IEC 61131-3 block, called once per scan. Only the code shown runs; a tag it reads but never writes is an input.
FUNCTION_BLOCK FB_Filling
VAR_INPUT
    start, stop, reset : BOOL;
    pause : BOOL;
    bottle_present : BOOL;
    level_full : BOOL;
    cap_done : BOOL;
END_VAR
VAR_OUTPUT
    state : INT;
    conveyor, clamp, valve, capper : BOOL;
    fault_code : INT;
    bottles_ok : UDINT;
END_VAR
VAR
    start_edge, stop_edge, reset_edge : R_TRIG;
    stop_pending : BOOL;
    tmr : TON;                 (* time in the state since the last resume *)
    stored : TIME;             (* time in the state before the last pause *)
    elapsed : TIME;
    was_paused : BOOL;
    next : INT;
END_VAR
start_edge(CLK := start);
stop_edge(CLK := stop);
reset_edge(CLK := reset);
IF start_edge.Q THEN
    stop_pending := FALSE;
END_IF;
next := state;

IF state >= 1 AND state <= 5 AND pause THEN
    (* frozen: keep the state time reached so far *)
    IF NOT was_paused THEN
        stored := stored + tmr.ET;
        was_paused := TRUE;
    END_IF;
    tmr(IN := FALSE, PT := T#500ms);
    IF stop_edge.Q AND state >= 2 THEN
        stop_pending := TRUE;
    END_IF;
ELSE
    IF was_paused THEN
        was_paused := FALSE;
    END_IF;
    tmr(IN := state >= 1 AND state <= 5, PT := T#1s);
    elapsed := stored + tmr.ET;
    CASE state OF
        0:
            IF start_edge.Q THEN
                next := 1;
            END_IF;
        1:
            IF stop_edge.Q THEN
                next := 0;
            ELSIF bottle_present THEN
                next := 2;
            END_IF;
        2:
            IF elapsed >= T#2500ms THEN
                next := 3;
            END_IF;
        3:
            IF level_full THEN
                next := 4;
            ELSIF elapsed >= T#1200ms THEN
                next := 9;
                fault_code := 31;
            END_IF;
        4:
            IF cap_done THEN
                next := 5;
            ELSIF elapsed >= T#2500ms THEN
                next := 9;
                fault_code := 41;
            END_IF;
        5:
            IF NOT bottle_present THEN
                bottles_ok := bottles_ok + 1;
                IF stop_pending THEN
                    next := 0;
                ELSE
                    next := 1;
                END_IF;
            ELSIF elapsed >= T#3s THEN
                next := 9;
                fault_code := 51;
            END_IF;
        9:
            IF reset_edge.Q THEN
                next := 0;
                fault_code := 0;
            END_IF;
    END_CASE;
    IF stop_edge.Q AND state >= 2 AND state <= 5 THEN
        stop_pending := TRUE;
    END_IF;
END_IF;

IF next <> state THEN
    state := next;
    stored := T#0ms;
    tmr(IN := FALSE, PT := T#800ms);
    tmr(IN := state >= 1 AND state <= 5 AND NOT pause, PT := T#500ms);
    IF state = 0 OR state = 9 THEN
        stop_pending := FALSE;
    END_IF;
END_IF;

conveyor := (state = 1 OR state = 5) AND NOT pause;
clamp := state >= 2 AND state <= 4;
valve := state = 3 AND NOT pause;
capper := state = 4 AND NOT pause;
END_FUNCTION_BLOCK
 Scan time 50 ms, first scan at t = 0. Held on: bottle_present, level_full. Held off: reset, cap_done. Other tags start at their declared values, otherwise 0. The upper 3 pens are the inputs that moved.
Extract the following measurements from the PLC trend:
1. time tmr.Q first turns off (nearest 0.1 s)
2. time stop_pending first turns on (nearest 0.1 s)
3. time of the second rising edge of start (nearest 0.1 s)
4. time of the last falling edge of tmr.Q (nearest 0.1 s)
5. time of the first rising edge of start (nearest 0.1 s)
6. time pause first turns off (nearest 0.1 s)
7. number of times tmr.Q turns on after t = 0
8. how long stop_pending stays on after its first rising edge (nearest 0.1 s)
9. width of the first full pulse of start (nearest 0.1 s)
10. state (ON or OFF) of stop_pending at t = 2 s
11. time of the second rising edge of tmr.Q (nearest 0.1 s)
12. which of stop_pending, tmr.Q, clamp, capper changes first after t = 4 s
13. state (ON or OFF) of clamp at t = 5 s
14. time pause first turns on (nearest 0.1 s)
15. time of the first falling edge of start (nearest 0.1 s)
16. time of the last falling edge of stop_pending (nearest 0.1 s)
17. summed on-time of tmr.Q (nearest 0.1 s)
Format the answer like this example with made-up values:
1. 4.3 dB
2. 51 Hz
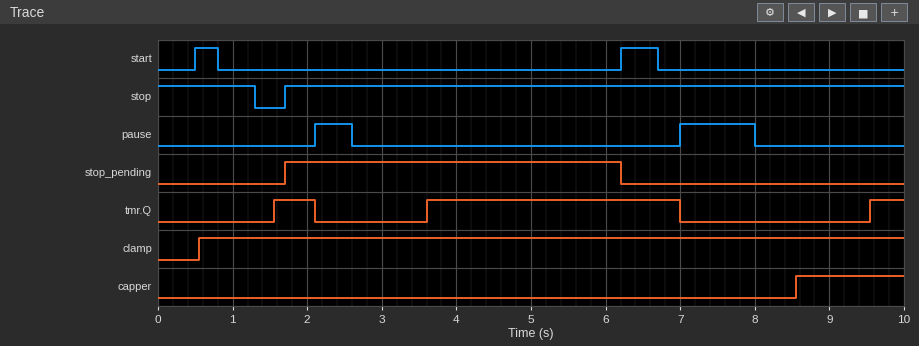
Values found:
1. 2.1 s
2. 1.7 s
3. 6.2 s
4. 7.0 s
5. 0.5 s
6. 2.6 s
7. 3
8. 4.5 s
9. 0.3 s
10. ON
11. 3.6 s
12. stop_pending
13. ON
14. 2.1 s
15. 0.8 s
16. 6.2 s
17. 4.4 s
